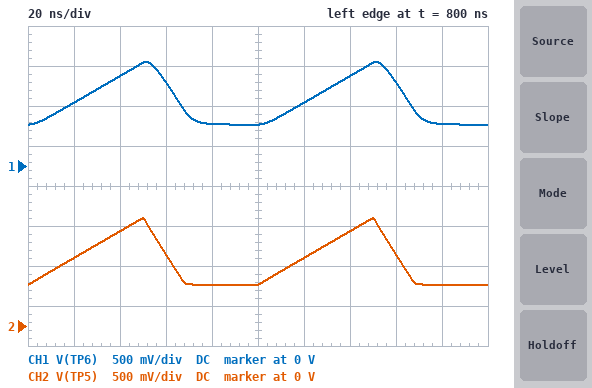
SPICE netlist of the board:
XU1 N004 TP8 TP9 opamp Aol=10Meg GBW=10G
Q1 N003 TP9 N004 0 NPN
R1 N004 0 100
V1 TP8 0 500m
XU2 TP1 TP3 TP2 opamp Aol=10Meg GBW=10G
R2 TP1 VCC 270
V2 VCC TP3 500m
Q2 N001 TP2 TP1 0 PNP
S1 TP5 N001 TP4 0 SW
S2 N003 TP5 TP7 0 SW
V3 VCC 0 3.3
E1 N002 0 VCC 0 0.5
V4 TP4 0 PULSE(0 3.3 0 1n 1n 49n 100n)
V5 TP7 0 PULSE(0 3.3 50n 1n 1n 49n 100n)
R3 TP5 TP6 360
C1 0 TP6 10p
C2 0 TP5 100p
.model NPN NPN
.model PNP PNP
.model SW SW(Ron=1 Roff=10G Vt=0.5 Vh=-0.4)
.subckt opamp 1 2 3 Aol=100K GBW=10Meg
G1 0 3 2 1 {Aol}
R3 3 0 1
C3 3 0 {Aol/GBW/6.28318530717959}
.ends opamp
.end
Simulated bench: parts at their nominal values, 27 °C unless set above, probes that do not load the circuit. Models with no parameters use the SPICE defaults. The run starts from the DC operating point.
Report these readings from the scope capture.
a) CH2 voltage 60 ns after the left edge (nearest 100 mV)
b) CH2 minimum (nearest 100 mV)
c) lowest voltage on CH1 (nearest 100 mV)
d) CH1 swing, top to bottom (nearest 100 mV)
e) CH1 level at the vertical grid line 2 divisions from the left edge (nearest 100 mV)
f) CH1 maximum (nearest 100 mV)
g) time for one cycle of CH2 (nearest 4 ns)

900 mV
500 mV
500 mV
800 mV
1.1 V
1.3 V
100 ns
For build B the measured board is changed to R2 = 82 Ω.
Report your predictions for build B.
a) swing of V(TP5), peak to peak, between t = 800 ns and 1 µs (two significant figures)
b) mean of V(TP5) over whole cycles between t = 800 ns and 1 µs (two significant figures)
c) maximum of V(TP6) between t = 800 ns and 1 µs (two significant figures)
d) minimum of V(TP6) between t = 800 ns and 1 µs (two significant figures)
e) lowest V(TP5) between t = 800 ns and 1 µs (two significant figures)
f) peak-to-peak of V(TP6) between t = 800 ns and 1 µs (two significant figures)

2.2 V
1.8 V
2.8 V
650 mV
540 mV
2.1 V
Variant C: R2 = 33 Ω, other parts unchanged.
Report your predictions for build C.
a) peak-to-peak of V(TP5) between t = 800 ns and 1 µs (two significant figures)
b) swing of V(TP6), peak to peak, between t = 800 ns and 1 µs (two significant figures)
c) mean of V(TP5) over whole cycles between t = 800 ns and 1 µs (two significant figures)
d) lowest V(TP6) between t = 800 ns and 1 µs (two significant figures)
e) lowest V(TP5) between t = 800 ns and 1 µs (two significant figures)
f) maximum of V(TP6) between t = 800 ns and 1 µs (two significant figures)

2.2 V
2.1 V
2.0 V
680 mV
550 mV
2.8 V
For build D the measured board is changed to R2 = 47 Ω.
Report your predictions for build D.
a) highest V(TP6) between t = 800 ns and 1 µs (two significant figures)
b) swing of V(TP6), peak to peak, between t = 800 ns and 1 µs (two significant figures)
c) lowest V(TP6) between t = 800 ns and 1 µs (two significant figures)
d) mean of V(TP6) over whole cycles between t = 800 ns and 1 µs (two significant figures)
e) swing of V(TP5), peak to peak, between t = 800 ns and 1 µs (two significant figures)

2.8 V
2.1 V
670 mV
2.0 V
2.2 V
